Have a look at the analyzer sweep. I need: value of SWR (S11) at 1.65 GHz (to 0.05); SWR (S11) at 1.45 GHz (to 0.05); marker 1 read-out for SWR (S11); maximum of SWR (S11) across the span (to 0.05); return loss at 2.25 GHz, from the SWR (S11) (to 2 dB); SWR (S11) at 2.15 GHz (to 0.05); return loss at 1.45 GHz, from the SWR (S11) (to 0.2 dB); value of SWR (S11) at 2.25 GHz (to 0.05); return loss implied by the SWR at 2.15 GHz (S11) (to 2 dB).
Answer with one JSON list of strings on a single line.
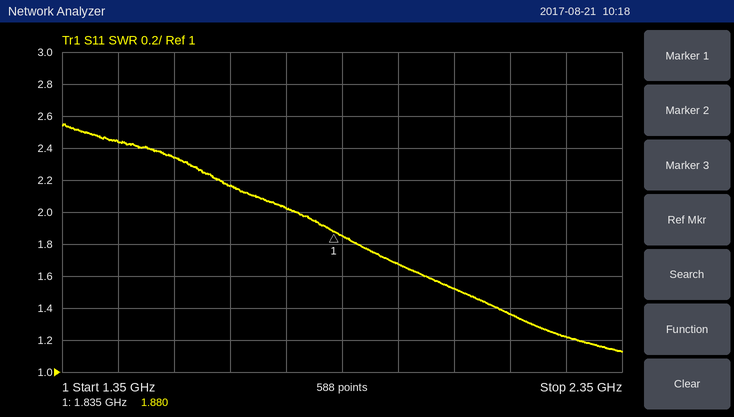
["2.15", "2.45", "1.880", "2.55", "20 dB", "1.35", "7.6 dB", "1.20", "16 dB"]
